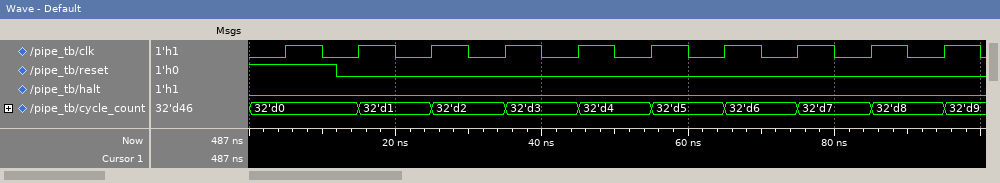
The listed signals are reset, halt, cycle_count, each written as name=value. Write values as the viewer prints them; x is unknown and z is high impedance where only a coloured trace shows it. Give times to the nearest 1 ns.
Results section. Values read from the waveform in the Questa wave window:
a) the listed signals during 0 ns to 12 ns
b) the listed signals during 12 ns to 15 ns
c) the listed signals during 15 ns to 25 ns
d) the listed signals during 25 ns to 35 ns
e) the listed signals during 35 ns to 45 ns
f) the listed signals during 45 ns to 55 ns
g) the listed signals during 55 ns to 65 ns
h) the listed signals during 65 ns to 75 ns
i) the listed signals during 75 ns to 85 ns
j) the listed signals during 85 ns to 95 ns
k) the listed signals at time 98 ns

reset=1, halt=0, cycle_count=32'd0
reset=0, halt=0, cycle_count=32'd0
reset=0, halt=0, cycle_count=32'd1
reset=0, halt=0, cycle_count=32'd2
reset=0, halt=0, cycle_count=32'd3
reset=0, halt=0, cycle_count=32'd4
reset=0, halt=0, cycle_count=32'd5
reset=0, halt=0, cycle_count=32'd6
reset=0, halt=0, cycle_count=32'd7
reset=0, halt=0, cycle_count=32'd8
reset=0, halt=0, cycle_count=32'd9
